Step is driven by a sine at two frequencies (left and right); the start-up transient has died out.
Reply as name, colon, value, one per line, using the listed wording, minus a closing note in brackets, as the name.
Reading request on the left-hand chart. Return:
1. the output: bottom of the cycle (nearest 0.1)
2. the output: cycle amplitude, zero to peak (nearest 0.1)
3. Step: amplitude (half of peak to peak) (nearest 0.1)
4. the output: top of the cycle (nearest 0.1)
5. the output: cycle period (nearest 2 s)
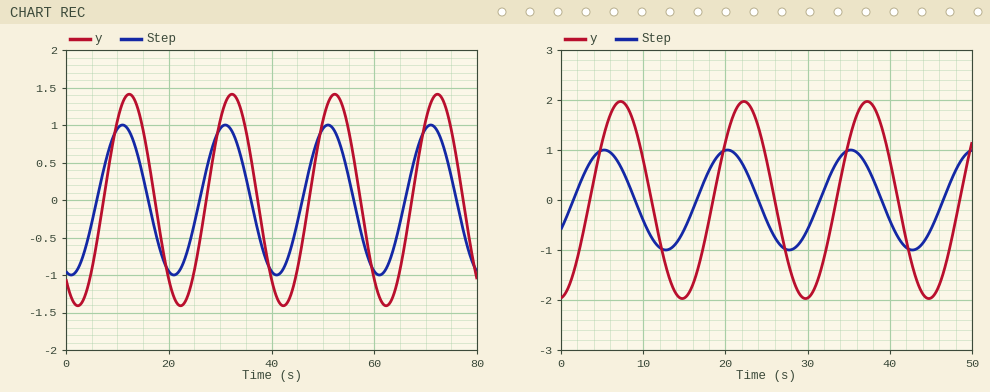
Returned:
the output: bottom of the cycle: -1.4
the output: cycle amplitude, zero to peak: 1.4
Step: amplitude (half of peak to peak): 1.0
the output: top of the cycle: 1.4
the output: cycle period: 20 s
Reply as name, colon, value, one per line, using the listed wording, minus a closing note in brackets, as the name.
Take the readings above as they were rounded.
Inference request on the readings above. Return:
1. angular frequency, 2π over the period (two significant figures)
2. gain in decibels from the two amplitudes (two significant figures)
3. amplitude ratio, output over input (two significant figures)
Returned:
angular frequency, 2π over the period: 0.31 rad/s
gain in decibels from the two amplitudes: 2.9 dB
amplitude ratio, output over input: 1.4
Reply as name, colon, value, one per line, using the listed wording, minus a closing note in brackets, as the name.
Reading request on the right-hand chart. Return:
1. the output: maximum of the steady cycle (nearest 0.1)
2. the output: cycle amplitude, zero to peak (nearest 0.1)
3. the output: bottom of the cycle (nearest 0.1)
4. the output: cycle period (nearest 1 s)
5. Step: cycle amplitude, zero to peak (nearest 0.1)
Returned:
the output: maximum of the steady cycle: 2.0
the output: cycle amplitude, zero to peak: 2.0
the output: bottom of the cycle: -2.0
the output: cycle period: 15 s
Step: cycle amplitude, zero to peak: 1.0
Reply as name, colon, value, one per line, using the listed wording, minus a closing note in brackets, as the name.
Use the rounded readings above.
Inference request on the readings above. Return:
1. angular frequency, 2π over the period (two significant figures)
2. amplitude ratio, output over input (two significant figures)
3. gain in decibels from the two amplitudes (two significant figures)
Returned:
angular frequency, 2π over the period: 0.42 rad/s
amplitude ratio, output over input: 2.0
gain in decibels from the two amplitudes: 6.0 dB
